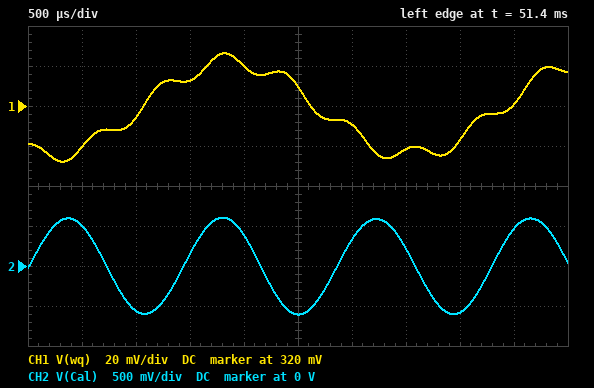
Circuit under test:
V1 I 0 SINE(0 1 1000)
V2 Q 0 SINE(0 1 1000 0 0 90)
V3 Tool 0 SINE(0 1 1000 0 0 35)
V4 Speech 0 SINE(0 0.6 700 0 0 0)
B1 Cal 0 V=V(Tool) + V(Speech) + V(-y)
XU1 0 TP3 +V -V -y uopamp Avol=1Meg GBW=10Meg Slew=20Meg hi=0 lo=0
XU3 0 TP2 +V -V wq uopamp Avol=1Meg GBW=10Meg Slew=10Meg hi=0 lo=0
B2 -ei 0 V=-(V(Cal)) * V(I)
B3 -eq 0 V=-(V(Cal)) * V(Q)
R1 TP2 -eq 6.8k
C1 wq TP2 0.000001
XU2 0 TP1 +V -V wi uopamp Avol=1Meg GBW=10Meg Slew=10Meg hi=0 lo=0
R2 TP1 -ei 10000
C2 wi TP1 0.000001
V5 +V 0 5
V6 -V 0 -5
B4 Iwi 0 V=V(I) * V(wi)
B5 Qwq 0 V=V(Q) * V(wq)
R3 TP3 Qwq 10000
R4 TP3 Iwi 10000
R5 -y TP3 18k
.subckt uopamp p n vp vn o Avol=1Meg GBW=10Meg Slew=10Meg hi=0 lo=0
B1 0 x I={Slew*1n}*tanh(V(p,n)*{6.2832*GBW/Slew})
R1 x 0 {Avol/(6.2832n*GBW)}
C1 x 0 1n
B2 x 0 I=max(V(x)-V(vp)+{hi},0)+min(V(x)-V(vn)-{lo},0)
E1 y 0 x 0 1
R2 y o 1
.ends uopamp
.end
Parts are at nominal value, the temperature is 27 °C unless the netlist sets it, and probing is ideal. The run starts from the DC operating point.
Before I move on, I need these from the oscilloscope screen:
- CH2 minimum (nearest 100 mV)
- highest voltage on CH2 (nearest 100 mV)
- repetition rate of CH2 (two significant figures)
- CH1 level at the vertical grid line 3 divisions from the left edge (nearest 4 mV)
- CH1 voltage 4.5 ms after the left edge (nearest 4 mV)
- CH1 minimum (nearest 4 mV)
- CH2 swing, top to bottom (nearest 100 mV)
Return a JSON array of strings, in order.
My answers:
["-600 mV", "600 mV", "700 Hz", "332 mV", "320 mV", "292 mV", "1.2 V"]
